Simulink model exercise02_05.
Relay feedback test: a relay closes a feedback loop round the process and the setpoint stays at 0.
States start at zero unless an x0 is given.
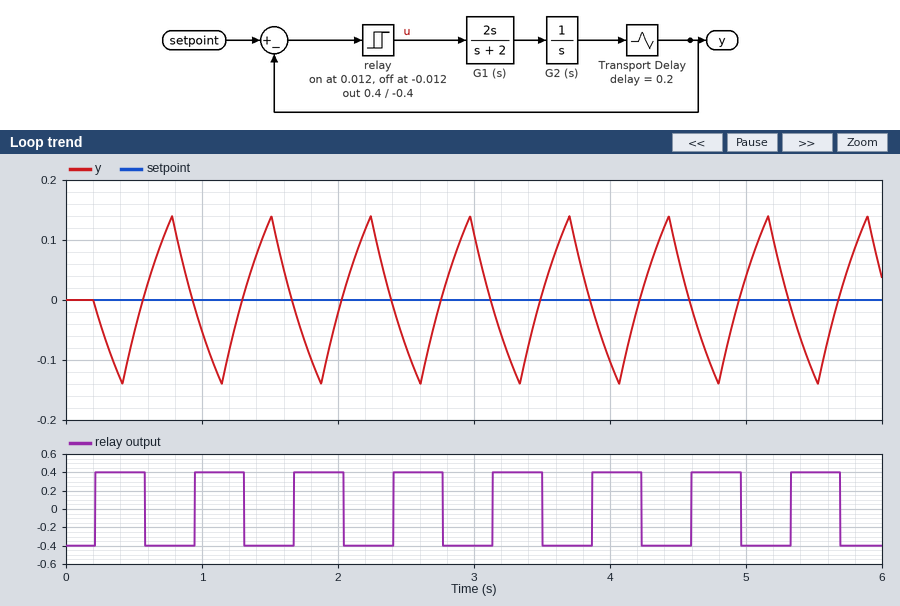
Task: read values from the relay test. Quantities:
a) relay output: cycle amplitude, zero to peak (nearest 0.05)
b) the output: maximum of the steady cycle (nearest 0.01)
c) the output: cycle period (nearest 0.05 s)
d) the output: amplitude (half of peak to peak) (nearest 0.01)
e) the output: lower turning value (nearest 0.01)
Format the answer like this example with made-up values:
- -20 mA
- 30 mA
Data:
- 0.40
- 0.14
- 0.75 s
- 0.14
- -0.14
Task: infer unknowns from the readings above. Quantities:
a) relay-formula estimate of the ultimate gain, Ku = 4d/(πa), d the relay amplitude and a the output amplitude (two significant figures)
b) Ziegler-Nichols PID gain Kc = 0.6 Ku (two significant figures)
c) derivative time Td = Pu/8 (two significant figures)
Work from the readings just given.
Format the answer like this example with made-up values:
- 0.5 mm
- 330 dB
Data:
- 3.6
- 2.2
- 0.094 s
